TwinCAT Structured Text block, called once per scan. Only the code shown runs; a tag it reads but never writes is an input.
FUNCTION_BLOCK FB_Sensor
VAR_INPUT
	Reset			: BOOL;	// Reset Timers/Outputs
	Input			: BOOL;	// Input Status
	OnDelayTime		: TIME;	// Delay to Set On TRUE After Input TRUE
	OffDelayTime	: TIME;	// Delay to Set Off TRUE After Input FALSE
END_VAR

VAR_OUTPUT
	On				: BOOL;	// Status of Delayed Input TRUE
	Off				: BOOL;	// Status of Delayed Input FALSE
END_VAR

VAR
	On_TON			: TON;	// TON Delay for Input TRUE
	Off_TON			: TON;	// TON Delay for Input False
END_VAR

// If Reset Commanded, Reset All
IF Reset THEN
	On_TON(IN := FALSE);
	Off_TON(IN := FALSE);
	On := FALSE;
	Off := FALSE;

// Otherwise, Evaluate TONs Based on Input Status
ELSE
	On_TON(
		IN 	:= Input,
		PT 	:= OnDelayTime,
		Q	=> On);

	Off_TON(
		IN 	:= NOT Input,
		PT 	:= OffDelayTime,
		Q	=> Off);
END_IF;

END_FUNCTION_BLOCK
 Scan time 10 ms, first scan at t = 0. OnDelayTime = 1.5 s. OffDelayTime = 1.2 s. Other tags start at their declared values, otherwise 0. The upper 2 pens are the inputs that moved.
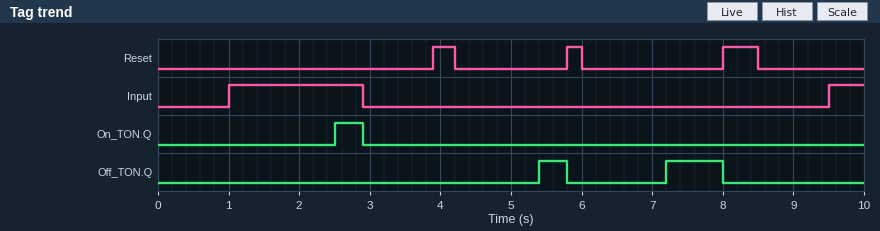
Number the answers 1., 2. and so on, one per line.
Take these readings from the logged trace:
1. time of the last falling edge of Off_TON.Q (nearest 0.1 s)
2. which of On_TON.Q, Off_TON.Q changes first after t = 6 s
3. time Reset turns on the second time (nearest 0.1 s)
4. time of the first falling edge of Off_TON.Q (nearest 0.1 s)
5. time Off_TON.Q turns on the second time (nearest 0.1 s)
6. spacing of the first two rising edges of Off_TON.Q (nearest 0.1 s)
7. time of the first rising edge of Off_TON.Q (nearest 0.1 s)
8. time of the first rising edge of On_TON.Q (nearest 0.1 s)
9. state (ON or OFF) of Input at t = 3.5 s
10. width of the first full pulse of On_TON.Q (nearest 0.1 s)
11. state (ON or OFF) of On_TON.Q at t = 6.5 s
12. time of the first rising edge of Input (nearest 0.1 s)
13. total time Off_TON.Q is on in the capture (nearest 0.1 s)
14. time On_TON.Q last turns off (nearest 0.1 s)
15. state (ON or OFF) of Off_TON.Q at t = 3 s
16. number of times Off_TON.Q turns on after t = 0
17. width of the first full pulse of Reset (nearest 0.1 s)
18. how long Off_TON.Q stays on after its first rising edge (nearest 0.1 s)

1. 8.0 s
2. Off_TON.Q
3. 5.8 s
4. 5.8 s
5. 7.2 s
6. 1.8 s
7. 5.4 s
8. 2.5 s
9. OFF
10. 0.4 s
11. OFF
12. 1.0 s
13. 1.2 s
14. 2.9 s
15. OFF
16. 2
17. 0.3 s
18. 0.4 s
